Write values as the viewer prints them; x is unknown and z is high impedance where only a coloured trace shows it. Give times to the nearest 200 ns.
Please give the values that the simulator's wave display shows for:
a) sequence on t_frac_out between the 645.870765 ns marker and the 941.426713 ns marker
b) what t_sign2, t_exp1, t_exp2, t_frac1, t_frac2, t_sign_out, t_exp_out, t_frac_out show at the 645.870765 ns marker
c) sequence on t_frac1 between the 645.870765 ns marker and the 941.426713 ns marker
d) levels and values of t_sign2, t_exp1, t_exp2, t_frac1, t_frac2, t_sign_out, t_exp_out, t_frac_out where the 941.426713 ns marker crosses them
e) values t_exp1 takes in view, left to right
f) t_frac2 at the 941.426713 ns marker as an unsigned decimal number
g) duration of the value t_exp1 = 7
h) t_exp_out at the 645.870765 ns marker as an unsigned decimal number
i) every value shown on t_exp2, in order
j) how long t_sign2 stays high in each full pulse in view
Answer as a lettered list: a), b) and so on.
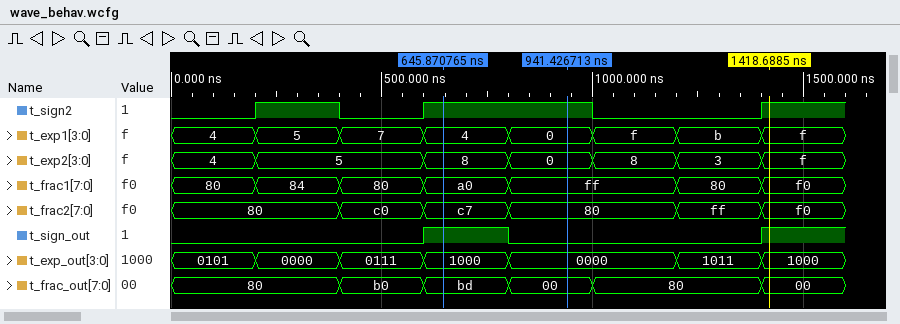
a) bd, 00
b) t_sign2=1, t_exp1=4, t_exp2=8, t_frac1=a0, t_frac2=c7, t_sign_out=1, t_exp_out=1000, t_frac_out=bd
c) a0, ff
d) t_sign2=1, t_exp1=0, t_exp2=0, t_frac1=ff, t_frac2=80, t_sign_out=0, t_exp_out=0000, t_frac_out=00
e) 4, 5, 7, 4, 0, f, b, f
f) 128
g) 200 ns
h) 8
i) 4, 5, 8, 0, 8, 3, f
j) 200 ns, 400 ns
